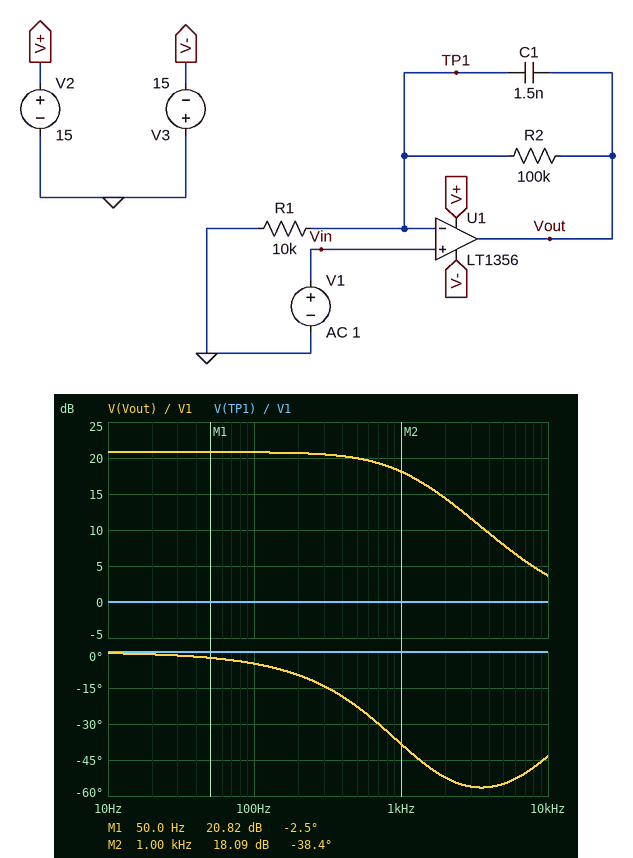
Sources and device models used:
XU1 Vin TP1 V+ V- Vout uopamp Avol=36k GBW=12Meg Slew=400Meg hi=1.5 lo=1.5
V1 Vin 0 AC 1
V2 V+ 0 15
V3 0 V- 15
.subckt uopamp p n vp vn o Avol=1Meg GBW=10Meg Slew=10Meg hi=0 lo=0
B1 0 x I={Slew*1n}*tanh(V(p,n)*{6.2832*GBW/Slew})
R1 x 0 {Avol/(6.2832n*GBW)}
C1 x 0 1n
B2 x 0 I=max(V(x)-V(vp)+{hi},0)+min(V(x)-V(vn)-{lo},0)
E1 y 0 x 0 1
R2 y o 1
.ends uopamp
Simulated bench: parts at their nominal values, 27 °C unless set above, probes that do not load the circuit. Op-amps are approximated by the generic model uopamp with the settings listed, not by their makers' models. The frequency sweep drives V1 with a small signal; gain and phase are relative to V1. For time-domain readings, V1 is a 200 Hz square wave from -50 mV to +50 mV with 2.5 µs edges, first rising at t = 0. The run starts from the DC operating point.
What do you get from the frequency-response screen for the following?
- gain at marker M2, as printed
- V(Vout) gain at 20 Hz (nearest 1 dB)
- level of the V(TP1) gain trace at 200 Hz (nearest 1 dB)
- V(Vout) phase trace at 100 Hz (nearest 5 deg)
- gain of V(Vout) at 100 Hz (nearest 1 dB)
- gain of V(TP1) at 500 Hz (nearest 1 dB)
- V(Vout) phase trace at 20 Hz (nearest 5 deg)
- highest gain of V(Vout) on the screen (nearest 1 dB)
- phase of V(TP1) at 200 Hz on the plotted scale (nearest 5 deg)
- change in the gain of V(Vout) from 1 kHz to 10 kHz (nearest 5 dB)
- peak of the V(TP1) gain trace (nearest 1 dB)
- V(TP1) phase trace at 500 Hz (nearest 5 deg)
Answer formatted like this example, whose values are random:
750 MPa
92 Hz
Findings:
18.09 dB
21 dB
0 dB
-5 deg
21 dB
0 dB
0 deg
21 dB
0 deg
-15 dB
0 dB
0 deg
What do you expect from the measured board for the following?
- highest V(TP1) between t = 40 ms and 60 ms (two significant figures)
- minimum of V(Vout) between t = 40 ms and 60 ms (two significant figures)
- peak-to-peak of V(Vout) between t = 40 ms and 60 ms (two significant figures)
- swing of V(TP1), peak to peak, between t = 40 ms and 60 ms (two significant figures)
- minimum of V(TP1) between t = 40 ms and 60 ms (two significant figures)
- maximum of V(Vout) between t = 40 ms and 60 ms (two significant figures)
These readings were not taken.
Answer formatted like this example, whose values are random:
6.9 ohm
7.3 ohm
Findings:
50 mV
-550 mV
1.1 V
100 mV
-50 mV
550 mV
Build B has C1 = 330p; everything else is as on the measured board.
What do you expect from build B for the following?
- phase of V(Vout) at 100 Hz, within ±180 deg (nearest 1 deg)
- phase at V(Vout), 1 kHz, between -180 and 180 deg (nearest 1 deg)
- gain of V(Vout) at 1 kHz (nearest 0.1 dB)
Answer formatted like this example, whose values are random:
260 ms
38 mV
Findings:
-1 deg
-11 deg
20.6 dB
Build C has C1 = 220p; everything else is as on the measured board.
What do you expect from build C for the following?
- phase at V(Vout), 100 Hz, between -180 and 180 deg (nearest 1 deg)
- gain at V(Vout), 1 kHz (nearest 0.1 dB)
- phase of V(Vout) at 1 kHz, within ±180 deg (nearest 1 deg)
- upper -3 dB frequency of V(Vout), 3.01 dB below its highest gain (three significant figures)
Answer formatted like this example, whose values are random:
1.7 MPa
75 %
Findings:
-1 deg
20.7 dB
-7 deg
7.25 kHz
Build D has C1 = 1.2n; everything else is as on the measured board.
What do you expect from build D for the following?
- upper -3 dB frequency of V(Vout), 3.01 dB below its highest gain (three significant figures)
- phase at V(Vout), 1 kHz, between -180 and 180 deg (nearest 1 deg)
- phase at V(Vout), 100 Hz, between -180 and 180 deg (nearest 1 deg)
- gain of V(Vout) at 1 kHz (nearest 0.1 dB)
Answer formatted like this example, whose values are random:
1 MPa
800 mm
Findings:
1.34 kHz
-33 deg
-4 deg
18.9 dB
